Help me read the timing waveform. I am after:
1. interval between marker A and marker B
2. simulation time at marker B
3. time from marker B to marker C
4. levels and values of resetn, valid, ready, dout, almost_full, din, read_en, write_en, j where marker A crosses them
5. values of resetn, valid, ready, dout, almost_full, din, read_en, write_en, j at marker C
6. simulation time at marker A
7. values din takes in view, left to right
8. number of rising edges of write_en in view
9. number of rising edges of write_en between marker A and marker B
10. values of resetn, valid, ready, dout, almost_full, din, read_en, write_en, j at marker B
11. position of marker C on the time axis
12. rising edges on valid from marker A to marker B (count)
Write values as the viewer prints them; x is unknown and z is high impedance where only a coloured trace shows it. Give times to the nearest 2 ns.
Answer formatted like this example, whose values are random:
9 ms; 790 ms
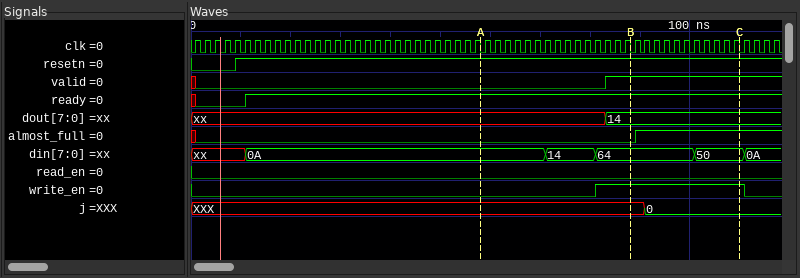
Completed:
30 ns; 88 ns; 22 ns; resetn=1, valid=0, ready=1, dout=xx, almost_full=0, din=0A, read_en=0, write_en=0, j=XXX; resetn=1, valid=1, ready=1, dout=14, almost_full=1, din=50, read_en=0, write_en=1, j=0; 58 ns; xx, 0A, 14, 64, 50, 0A; 1; 1; resetn=1, valid=1, ready=1, dout=14, almost_full=0, din=64, read_en=0, write_en=1, j=XXX; 110 ns; 1
